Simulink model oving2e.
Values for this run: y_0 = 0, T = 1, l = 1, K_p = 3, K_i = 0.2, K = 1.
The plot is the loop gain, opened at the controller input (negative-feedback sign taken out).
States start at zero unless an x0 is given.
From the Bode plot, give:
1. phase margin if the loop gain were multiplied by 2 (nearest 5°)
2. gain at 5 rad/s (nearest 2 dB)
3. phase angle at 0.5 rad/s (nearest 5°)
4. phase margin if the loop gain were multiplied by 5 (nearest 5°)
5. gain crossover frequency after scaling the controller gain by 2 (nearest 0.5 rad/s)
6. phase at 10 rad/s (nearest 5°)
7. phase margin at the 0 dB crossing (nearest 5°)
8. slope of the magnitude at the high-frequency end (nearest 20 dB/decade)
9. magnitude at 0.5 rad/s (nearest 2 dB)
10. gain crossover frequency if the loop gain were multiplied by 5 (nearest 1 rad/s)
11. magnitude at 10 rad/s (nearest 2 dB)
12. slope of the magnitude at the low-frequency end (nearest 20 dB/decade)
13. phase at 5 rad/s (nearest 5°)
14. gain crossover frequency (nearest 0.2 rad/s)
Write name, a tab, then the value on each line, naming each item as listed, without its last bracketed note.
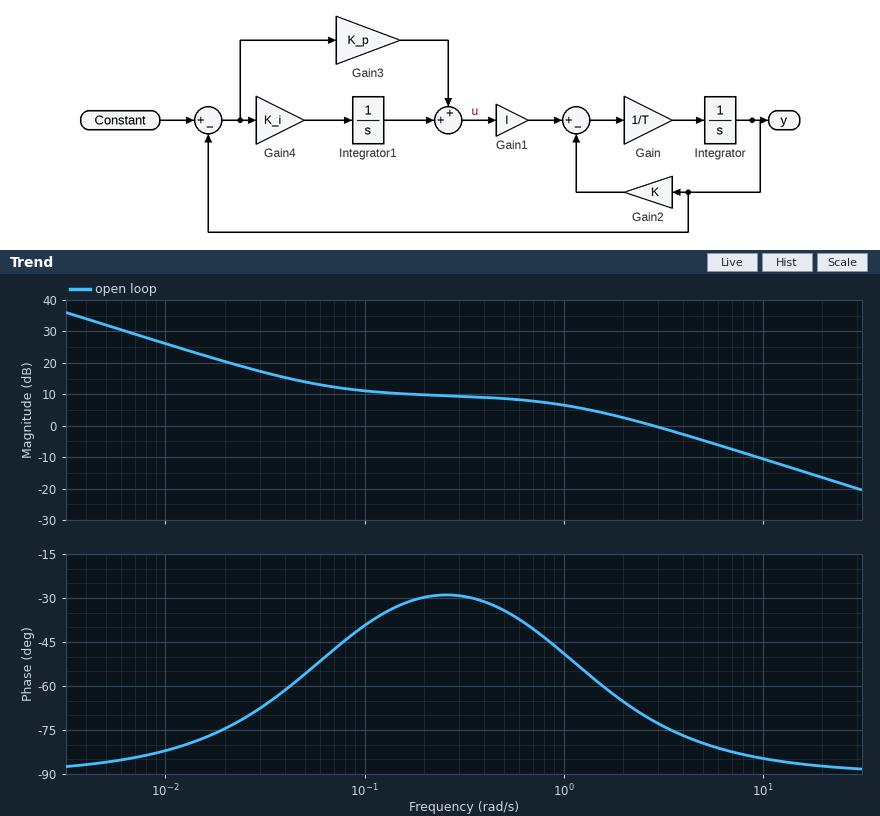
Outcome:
phase margin if the loop gain were multiplied by 2	100°
gain at 5 rad/s	-4 dB
phase angle at 0.5 rad/s	-35°
phase margin if the loop gain were multiplied by 5	95°
gain crossover frequency after scaling the controller gain by 2	6.0 rad/s
phase at 10 rad/s	-85°
phase margin at the 0 dB crossing	110°
slope of the magnitude at the high-frequency end	-20 dB/decade
magnitude at 0.5 rad/s	8 dB
gain crossover frequency if the loop gain were multiplied by 5	15 rad/s
magnitude at 10 rad/s	-10 dB
slope of the magnitude at the low-frequency end	-20 dB/decade
phase at 5 rad/s	-80°
gain crossover frequency	2.8 rad/s
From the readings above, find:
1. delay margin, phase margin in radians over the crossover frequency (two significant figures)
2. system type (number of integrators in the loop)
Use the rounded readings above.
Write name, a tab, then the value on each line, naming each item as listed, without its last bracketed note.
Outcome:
delay margin, phase margin in radians over the crossover frequency	0.69 s
system type	1
